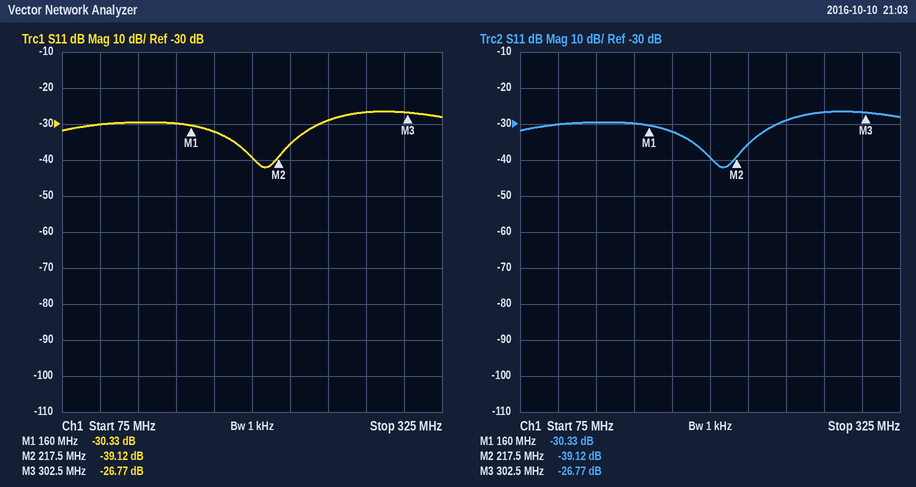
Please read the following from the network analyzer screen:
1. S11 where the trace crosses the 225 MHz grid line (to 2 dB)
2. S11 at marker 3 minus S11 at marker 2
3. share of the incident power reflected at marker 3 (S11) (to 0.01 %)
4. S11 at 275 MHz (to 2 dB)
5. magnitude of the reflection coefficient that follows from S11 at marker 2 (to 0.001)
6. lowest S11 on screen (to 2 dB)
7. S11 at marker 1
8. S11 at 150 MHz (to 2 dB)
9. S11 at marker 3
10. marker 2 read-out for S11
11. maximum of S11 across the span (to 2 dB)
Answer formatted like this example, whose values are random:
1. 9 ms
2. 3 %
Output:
1. -36 dB
2. 12.35 dB
3. 0.21 %
4. -26 dB
5. 0.011
6. -42 dB
7. -30.33 dB
8. -30 dB
9. -26.77 dB
10. -39.12 dB
11. -26 dB
